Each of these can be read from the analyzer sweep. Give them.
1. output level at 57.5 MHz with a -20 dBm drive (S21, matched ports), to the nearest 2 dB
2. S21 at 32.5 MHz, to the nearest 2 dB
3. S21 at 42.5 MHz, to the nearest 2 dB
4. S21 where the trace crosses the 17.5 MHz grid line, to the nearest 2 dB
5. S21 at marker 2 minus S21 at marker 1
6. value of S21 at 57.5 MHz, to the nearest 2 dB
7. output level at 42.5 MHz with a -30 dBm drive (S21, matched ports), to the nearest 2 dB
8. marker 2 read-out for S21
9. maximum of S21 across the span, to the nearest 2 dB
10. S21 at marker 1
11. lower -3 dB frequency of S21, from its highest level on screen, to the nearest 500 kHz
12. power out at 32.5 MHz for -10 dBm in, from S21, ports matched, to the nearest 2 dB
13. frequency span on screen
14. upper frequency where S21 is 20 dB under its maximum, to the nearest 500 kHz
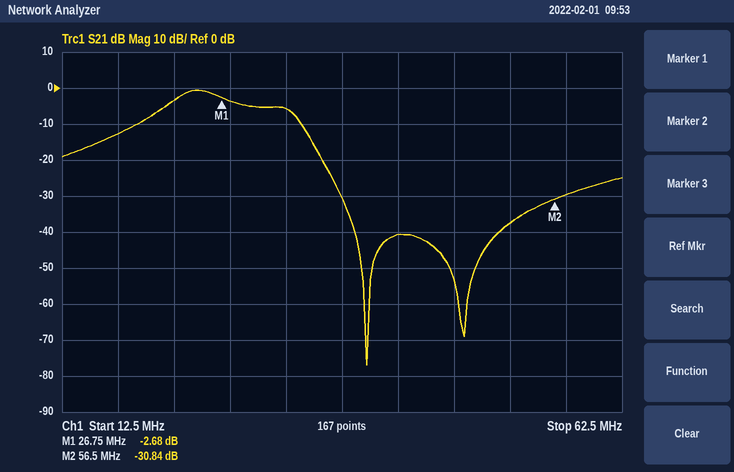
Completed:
-50 dBm
-6 dB
-40 dB
-12 dB
-28.16 dB
-30 dB
-70 dBm
-30.84 dB
0 dB
-2.68 dB
22.5 MHz
-16 dBm
50 MHz
36.0 MHz
